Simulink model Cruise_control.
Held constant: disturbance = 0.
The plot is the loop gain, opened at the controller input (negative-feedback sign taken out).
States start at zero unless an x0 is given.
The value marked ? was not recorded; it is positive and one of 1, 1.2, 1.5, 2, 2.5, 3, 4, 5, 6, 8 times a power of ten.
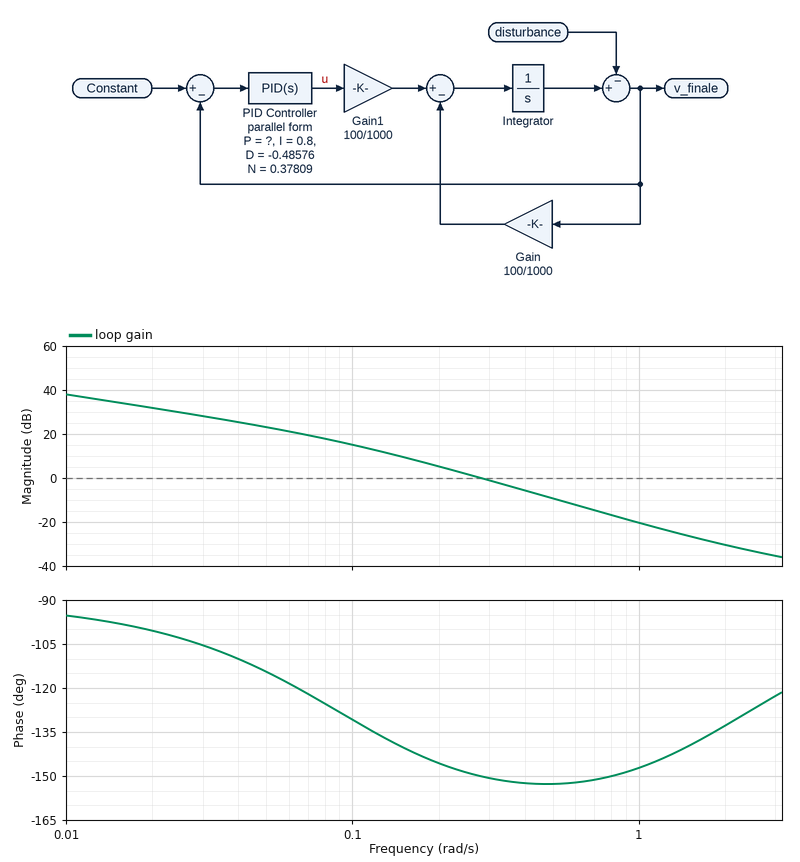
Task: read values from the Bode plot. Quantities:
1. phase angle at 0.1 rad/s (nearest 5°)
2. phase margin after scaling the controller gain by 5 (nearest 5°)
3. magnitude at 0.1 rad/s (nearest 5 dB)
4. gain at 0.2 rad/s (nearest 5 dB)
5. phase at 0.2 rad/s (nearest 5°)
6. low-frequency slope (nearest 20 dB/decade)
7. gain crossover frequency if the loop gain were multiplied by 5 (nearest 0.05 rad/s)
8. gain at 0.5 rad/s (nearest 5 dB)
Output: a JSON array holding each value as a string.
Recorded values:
["-130°", "30°", "15 dB", "5 dB", "-145°", "-20 dB/decade", "0.65 rad/s", "-10 dB"]
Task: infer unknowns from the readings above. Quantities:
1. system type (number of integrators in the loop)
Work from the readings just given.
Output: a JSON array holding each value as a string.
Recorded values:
["1"]
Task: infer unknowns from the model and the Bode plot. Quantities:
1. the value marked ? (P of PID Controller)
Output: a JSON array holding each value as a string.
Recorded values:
["0.6"]
